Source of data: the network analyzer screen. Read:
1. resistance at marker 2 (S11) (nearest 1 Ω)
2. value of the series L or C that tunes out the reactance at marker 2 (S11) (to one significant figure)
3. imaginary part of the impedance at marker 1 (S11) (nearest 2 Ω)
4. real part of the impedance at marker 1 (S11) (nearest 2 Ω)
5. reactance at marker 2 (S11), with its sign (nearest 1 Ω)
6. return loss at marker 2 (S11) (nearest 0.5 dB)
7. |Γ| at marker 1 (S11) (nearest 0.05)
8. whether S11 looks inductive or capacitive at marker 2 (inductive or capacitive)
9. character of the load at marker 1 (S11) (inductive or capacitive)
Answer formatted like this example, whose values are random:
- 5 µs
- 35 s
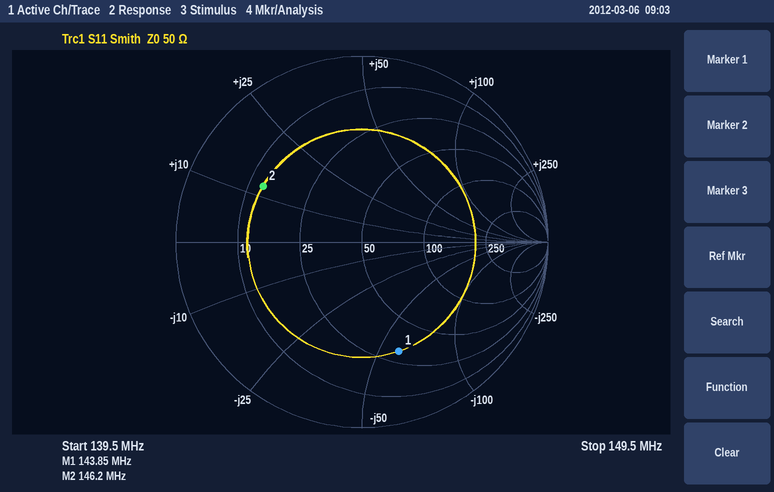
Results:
- 13 Ω
- 90 pF
- -60 Ω
- 32 Ω
- +12 Ω
- 4.5 dB
- 0.60
- inductive
- capacitive
